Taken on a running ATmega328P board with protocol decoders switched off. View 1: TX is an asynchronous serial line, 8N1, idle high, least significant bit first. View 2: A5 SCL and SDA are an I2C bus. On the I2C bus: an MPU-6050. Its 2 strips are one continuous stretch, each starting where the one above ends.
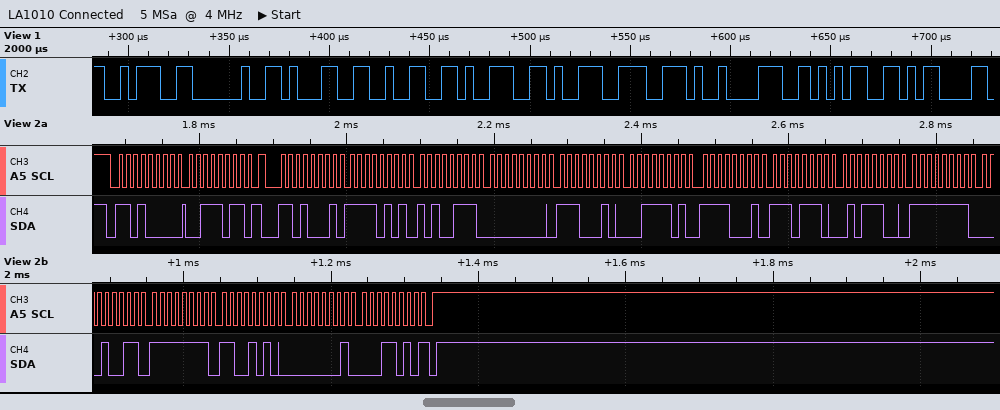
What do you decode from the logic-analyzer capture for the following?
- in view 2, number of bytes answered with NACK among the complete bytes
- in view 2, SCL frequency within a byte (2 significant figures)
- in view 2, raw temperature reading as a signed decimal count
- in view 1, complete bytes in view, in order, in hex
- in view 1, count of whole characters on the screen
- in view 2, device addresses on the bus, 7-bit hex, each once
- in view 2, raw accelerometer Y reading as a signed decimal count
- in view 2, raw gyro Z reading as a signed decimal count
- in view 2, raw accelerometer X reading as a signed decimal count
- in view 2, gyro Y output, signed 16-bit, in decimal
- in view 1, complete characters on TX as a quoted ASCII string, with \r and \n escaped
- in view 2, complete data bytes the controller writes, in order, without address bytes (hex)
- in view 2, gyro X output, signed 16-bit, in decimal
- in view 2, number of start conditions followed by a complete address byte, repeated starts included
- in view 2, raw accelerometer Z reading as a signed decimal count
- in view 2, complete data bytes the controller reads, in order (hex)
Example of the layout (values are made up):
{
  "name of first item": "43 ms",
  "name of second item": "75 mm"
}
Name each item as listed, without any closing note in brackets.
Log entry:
{
  "in view 2, number of bytes answered with NACK among the complete bytes": "1",
  "in view 2, SCL frequency within a byte": "100 kHz",
  "in view 2, raw temperature reading as a signed decimal count": "-4516",
  "in view 1, complete bytes in view, in order, in hex": "3A 20 31 32 39 39 2E 38 35 0D",
  "in view 1, count of whole characters on the screen": "10",
  "in view 2, device addresses on the bus, 7-bit hex, each once": "0x68",
  "in view 2, raw accelerometer Y reading as a signed decimal count": "226",
  "in view 2, raw gyro Z reading as a signed decimal count": "282",
  "in view 2, raw accelerometer X reading as a signed decimal count": "-2649",
  "in view 2, gyro Y output, signed 16-bit, in decimal": "-54",
  "in view 1, complete characters on TX as a quoted ASCII string, with \\r and \\n escaped": "\": 1299.85\\r\"",
  "in view 2, complete data bytes the controller writes, in order, without address bytes": "3B",
  "in view 2, gyro X output, signed 16-bit, in decimal": "-237",
  "in view 2, number of start conditions followed by a complete address byte, repeated starts included": "2",
  "in view 2, raw accelerometer Z reading as a signed decimal count": "15857",
  "in view 2, complete data bytes the controller reads, in order": "F5 A7 00 E2 3D F1 EE 5C FF 13 FF CA 01 1A"
}
